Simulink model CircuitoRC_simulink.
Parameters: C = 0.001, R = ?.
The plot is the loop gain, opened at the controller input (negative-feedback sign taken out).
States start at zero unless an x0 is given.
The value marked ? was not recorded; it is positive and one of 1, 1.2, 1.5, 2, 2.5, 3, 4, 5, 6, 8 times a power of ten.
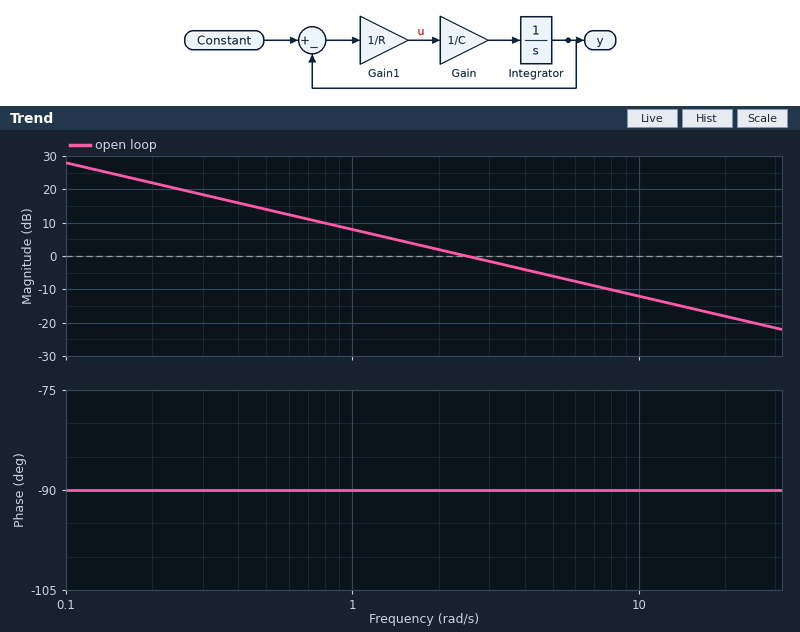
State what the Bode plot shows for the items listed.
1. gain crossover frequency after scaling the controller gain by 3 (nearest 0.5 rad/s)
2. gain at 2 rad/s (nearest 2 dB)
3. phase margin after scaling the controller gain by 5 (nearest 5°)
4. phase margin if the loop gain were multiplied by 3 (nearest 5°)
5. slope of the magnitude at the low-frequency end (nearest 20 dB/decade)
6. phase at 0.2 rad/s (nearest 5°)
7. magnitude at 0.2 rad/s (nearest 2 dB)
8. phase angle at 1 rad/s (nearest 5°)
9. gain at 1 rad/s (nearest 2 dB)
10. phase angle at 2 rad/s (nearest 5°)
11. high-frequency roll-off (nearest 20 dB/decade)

7.5 rad/s
2 dB
90°
90°
-20 dB/decade
-90°
22 dB
-90°
8 dB
-90°
-20 dB/decade
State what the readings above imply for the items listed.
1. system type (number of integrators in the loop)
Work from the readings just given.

1
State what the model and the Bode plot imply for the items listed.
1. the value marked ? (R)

400
